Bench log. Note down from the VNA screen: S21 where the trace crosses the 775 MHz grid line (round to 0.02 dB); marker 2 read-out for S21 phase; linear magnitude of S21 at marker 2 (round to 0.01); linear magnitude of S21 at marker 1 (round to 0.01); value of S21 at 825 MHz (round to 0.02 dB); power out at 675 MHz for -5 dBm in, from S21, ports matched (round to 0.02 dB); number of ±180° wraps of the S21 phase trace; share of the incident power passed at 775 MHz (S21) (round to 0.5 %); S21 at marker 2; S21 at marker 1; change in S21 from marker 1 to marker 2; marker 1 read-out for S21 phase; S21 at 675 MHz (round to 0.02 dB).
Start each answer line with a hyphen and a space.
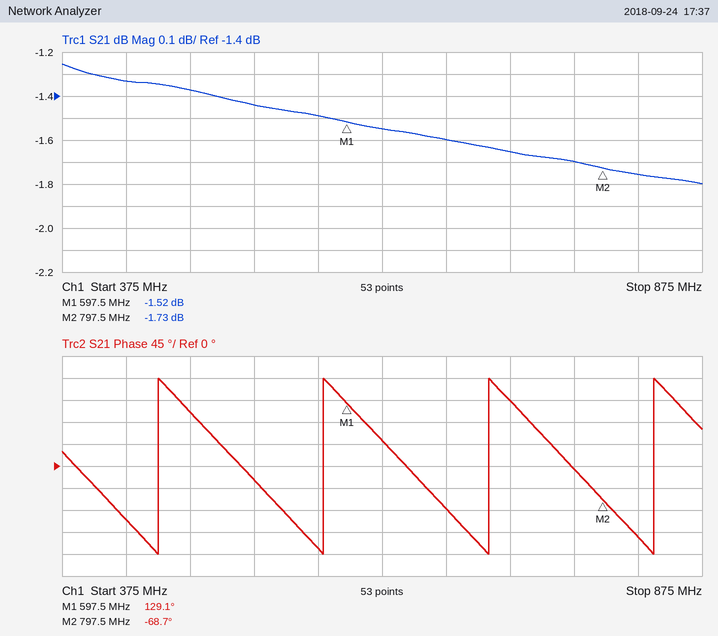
- -1.70 dB
- -68.7°
- 0.82
- 0.84
- -1.76 dB
- -6.60 dBm
- 4
- 67.5 %
- -1.73 dB
- -1.52 dB
- -0.21 dB
- 129.1°
- -1.60 dB
